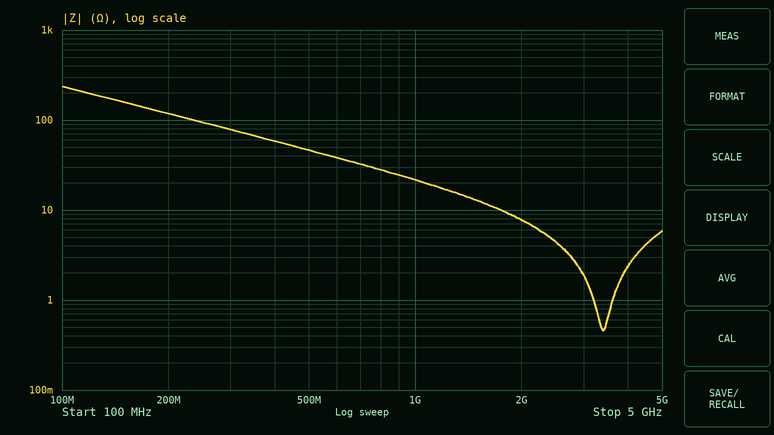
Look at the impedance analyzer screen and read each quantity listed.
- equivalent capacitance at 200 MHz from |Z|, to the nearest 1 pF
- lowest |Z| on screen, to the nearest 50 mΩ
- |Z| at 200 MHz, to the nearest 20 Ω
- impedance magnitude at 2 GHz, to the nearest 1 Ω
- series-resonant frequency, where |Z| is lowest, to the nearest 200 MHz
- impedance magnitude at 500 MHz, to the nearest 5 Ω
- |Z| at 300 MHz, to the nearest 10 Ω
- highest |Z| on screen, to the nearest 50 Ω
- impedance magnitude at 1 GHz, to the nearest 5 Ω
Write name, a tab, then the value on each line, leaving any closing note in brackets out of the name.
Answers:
equivalent capacitance at 200 MHz from |Z|, to the nearest 1 pF	7 pF
lowest |Z| on screen, to the nearest 50 mΩ	450 mΩ
|Z| at 200 MHz, to the nearest 20 Ω	120 Ω
impedance magnitude at 2 GHz, to the nearest 1 Ω	8 Ω
series-resonant frequency, where |Z| is lowest, to the nearest 200 MHz	3.4 GHz
impedance magnitude at 500 MHz, to the nearest 5 Ω	45 Ω
|Z| at 300 MHz, to the nearest 10 Ω	80 Ω
highest |Z| on screen, to the nearest 50 Ω	250 Ω
impedance magnitude at 1 GHz, to the nearest 5 Ω	20 Ω
